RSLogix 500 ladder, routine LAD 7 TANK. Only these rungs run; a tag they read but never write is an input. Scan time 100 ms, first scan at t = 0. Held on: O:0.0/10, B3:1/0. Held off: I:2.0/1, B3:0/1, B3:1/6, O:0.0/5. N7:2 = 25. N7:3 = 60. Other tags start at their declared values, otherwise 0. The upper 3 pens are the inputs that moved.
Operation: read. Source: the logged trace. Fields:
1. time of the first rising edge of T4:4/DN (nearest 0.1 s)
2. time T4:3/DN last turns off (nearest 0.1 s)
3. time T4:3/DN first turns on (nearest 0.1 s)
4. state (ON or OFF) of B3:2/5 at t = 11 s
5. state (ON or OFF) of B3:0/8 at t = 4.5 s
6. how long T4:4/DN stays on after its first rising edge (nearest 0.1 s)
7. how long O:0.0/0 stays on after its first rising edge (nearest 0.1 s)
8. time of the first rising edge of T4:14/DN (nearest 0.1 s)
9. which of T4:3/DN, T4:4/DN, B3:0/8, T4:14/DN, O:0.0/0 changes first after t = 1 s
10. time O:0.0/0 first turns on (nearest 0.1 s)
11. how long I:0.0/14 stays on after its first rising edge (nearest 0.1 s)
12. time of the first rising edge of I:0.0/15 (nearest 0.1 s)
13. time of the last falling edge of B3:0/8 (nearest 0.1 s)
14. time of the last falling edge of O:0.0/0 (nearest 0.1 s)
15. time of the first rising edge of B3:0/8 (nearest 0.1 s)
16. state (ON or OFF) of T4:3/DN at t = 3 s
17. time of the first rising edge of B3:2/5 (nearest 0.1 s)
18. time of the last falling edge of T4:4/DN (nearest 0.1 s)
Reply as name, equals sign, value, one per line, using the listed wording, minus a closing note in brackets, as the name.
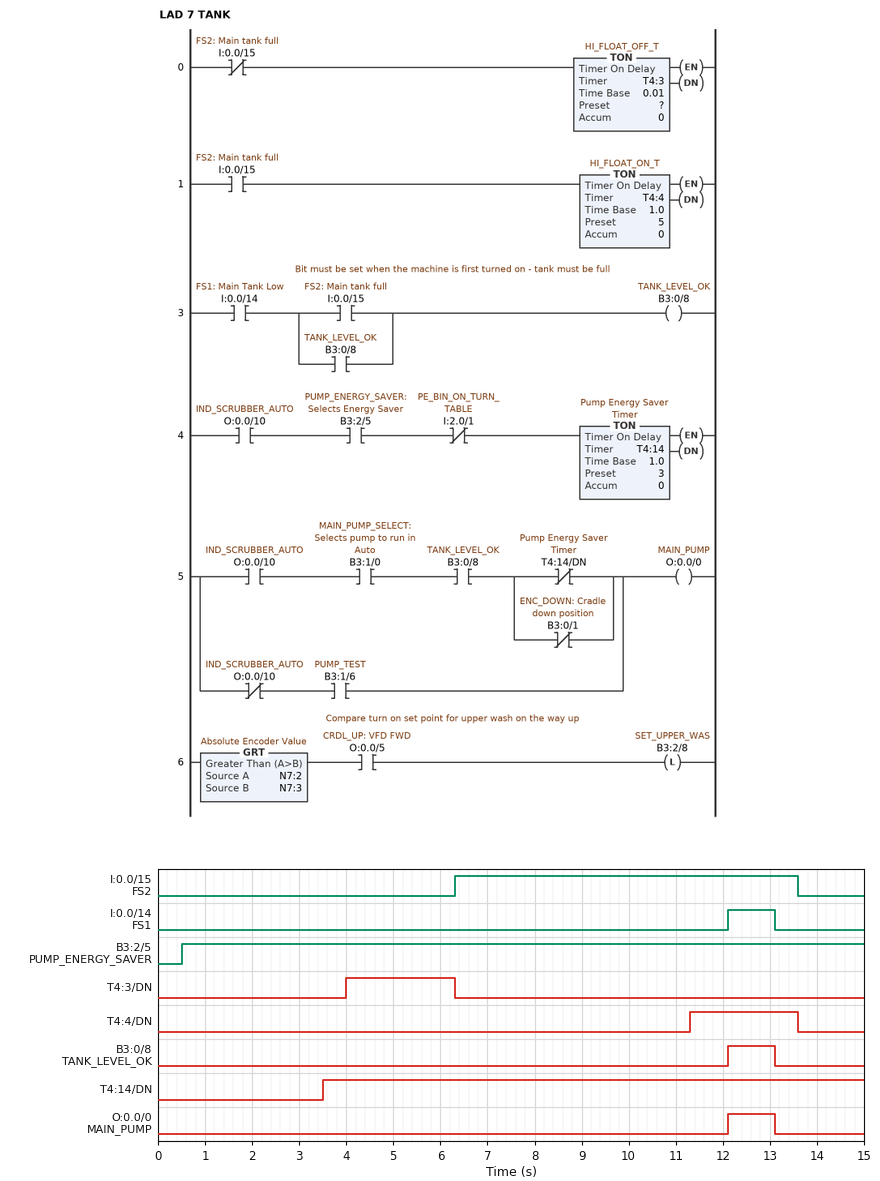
time of the first rising edge of T4:4/DN = 11.3 s
time T4:3/DN last turns off = 6.3 s
time T4:3/DN first turns on = 4.0 s
state (ON or OFF) of B3:2/5 at t = 11 s = ON
state (ON or OFF) of B3:0/8 at t = 4.5 s = OFF
how long T4:4/DN stays on after its first rising edge = 2.3 s
how long O:0.0/0 stays on after its first rising edge = 1.0 s
time of the first rising edge of T4:14/DN = 3.5 s
which of T4:3/DN, T4:4/DN, B3:0/8, T4:14/DN, O:0.0/0 changes first after t = 1 s = T4:14/DN
time O:0.0/0 first turns on = 12.1 s
how long I:0.0/14 stays on after its first rising edge = 1.0 s
time of the first rising edge of I:0.0/15 = 6.3 s
time of the last falling edge of B3:0/8 = 13.1 s
time of the last falling edge of O:0.0/0 = 13.1 s
time of the first rising edge of B3:0/8 = 12.1 s
state (ON or OFF) of T4:3/DN at t = 3 s = OFF
time of the first rising edge of B3:2/5 = 0.5 s
time of the last falling edge of T4:4/DN = 13.6 s
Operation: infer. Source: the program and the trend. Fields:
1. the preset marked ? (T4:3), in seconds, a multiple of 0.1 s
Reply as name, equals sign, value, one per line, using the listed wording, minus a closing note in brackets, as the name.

the preset marked ? (T4:3), in seconds, a multiple of 0.1 s = 4.0 s
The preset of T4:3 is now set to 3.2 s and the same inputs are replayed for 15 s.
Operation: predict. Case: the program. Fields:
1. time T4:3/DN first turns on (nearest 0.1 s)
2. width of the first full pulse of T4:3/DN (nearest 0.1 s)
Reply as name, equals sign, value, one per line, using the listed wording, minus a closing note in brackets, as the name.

time T4:3/DN first turns on = 3.2 s
width of the first full pulse of T4:3/DN = 3.1 s
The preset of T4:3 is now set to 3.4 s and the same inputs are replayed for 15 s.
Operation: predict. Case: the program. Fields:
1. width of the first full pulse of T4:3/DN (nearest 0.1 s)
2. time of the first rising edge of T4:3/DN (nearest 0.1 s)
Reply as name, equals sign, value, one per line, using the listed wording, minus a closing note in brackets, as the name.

width of the first full pulse of T4:3/DN = 2.9 s
time of the first rising edge of T4:3/DN = 3.4 s
